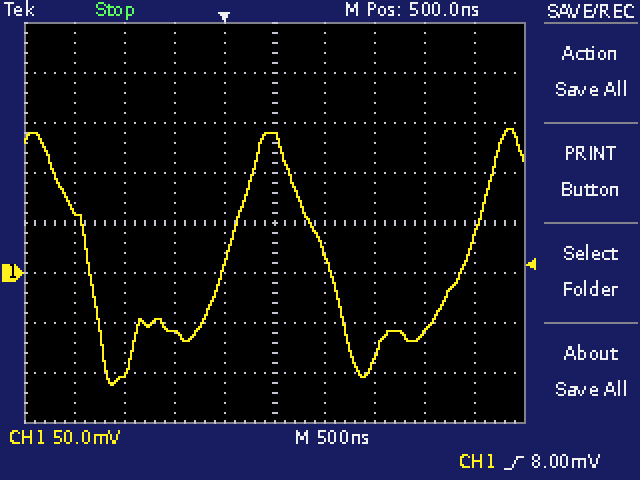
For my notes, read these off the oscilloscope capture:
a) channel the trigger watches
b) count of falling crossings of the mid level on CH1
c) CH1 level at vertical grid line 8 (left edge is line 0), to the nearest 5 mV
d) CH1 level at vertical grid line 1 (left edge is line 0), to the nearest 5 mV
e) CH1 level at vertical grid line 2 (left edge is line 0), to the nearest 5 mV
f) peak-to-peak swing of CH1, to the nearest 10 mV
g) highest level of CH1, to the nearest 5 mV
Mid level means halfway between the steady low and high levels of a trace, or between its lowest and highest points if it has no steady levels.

CH1
2
-60 mV
65 mV
-100 mV
260 mV
145 mV
